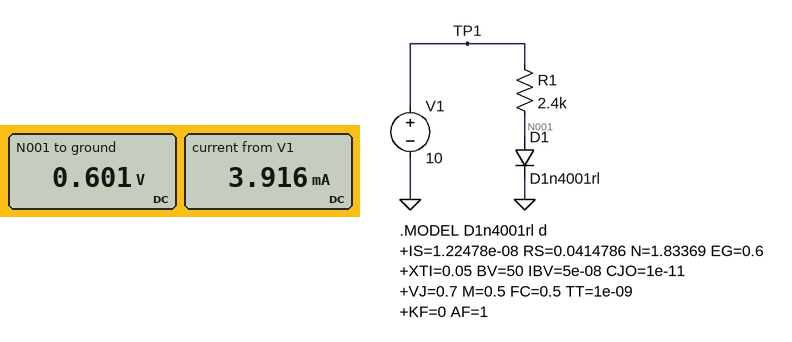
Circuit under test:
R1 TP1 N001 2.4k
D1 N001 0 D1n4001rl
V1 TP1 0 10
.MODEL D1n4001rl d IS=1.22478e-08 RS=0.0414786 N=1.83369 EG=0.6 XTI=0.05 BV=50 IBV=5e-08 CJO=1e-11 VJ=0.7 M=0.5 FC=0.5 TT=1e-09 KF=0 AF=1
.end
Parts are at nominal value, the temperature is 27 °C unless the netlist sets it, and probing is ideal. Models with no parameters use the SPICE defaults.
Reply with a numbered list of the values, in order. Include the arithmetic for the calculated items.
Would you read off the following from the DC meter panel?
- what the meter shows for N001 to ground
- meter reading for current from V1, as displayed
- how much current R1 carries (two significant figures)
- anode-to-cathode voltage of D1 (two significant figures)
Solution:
1. 0.601 V
2. 3.916 mA
3. (10 V - 601 mV) / 2.4 kΩ = 3.9 mA
4. 601 mV = 600 mV
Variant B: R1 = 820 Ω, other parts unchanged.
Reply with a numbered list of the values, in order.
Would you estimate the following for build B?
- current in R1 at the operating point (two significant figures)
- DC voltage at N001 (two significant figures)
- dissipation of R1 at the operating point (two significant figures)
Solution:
1. 11 mA
2. 650 mV
3. 110 mW
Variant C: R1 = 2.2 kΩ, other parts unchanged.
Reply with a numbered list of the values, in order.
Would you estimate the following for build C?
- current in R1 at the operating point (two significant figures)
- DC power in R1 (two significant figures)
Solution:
1. 4.3 mA
2. 40 mW
